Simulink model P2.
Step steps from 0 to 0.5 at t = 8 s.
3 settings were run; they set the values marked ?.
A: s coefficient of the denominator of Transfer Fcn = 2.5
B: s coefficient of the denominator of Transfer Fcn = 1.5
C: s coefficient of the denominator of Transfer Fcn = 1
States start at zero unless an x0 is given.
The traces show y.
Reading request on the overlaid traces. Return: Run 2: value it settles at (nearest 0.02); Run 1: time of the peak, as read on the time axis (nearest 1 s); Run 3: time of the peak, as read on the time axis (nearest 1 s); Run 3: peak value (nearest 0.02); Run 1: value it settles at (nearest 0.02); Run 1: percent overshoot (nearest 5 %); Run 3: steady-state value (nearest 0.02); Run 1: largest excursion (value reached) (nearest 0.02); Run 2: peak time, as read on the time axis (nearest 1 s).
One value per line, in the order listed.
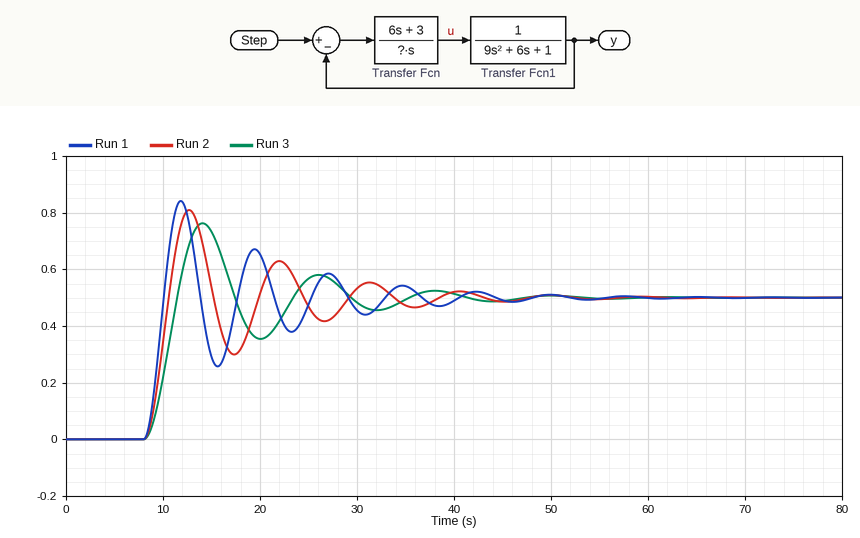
0.50
12 s
14 s
0.76
0.50
70 %
0.50
0.84
13 s
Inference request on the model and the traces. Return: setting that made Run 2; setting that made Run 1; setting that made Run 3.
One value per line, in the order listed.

B
C
A
